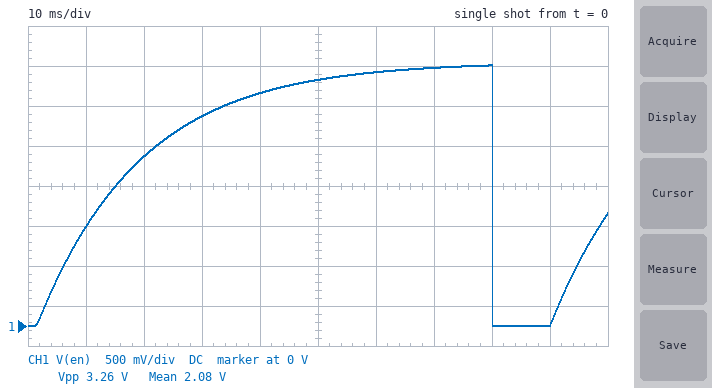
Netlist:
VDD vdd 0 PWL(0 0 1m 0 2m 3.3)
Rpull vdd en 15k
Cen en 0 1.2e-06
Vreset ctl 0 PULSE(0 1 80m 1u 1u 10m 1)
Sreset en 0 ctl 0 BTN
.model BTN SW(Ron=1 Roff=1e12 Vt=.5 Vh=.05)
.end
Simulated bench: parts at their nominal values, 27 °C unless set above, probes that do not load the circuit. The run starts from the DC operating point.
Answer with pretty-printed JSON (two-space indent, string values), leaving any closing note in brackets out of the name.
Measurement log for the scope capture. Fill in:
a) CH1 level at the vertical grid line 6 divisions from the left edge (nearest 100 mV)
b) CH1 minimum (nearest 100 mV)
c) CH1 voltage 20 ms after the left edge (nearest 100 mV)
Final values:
{
  "CH1 level at the vertical grid line 6 divisions from the left edge": "3.2 V",
  "CH1 minimum": "0 V",
  "CH1 voltage 20 ms after the left edge": "2.1 V"
}
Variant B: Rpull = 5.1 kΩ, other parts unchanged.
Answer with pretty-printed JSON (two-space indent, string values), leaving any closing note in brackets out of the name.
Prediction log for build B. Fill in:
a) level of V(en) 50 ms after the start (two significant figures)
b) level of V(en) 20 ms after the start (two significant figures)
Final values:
{
  "level of V(en) 50 ms after the start": "3.3 V",
  "level of V(en) 20 ms after the start": "3.1 V"
}
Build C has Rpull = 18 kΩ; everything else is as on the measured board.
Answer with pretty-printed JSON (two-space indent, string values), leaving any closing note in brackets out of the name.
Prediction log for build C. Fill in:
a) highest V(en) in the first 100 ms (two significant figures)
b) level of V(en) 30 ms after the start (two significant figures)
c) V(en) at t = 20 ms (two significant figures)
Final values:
{
  "highest V(en) in the first 100 ms": "3.2 V",
  "level of V(en) 30 ms after the start": "2.4 V",
  "V(en) at t = 20 ms": "1.9 V"
}
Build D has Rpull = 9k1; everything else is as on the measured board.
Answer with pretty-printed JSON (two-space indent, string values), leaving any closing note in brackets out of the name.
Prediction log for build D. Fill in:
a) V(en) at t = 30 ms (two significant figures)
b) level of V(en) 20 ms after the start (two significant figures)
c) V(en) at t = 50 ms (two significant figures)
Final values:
{
  "V(en) at t = 30 ms": "3.1 V",
  "level of V(en) 20 ms after the start": "2.7 V",
  "V(en) at t = 50 ms": "3.3 V"
}
